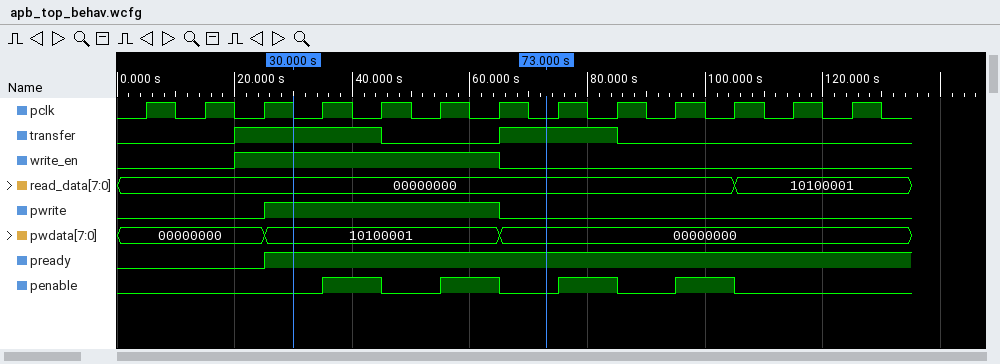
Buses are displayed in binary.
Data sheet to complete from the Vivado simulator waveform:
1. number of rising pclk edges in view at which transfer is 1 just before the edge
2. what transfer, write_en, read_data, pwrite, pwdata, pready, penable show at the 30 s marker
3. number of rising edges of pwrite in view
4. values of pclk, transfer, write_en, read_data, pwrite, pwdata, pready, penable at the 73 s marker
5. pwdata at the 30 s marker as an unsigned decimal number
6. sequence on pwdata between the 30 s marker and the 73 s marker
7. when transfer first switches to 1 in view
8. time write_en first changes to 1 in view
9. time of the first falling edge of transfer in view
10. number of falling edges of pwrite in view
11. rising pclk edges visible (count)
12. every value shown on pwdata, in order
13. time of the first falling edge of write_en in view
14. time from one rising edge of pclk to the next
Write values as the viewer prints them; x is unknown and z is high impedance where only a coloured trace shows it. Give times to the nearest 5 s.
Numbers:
5
transfer=1, write_en=1, read_data=00000000, pwrite=1, pwdata=10100001, pready=1, penable=0
1
pclk=0, transfer=1, write_en=0, read_data=00000000, pwrite=0, pwdata=00000000, pready=1, penable=0
161
10100001, 00000000
20 s
20 s
45 s
1
13
00000000, 10100001, 00000000
65 s
10 s
